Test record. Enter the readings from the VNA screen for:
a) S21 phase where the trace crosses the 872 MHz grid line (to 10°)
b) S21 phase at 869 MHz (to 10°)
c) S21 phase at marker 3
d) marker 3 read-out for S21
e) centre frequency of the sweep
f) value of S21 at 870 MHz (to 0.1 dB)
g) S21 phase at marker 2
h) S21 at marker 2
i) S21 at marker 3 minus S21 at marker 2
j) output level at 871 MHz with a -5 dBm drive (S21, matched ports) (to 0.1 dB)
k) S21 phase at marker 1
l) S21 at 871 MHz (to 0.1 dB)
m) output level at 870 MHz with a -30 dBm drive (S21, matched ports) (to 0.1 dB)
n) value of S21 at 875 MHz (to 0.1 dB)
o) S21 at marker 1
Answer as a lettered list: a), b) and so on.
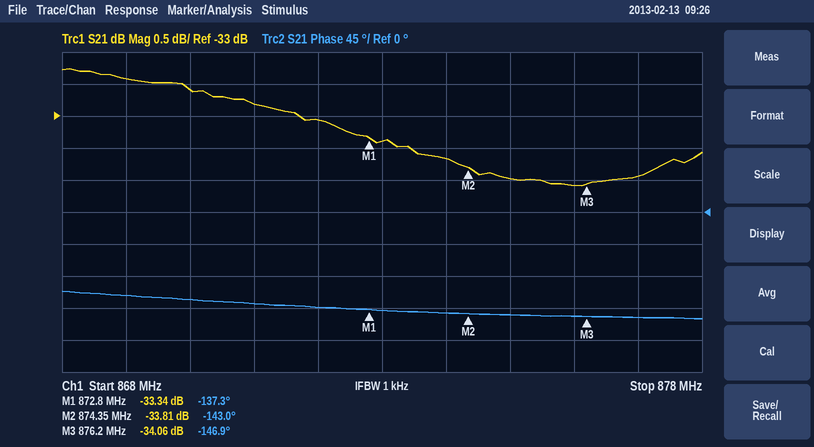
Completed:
a) -130°
b) -120°
c) -146.9°
d) -34.06 dB
e) 873 MHz
f) -32.6 dB
g) -143.0°
h) -33.81 dB
i) -0.25 dB
j) -37.8 dBm
k) -137.3°
l) -32.8 dB
m) -62.6 dBm
n) -34.0 dB
o) -33.34 dB
